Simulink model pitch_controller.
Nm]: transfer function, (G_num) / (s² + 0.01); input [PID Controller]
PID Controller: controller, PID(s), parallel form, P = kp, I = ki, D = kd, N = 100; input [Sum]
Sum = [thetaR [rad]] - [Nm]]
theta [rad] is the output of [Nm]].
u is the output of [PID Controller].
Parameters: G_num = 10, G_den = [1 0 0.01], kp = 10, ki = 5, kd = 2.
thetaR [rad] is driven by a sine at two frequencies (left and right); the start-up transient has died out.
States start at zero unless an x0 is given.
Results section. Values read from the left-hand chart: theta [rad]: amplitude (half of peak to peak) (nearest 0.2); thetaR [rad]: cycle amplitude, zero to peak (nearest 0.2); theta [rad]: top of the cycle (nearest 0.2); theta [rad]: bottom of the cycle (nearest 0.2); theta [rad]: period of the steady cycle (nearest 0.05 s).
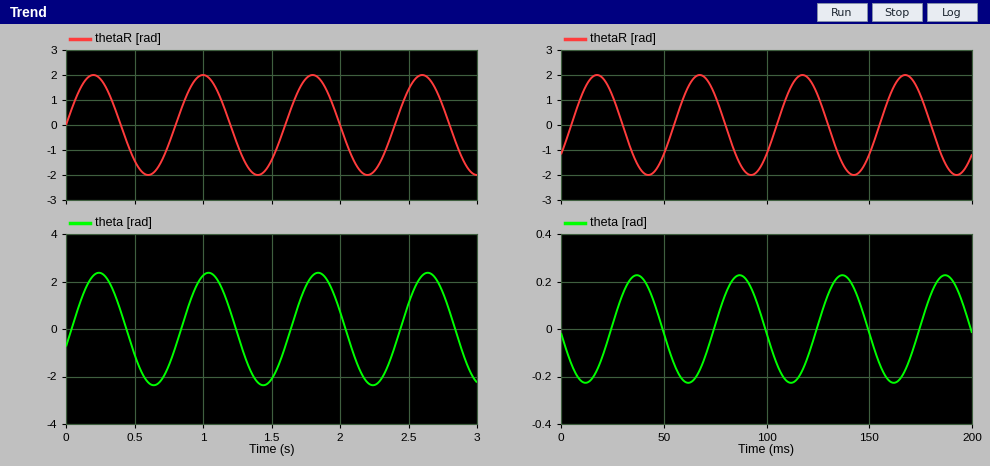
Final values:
2.4
2.0
2.4
-2.4
0.80 s
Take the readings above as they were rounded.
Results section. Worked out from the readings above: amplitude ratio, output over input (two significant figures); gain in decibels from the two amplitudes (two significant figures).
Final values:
1.2
1.6 dB
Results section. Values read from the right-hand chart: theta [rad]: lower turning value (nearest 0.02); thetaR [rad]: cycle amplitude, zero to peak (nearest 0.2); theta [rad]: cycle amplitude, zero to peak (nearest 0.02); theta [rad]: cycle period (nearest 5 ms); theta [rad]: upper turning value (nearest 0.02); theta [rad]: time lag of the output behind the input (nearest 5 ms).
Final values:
-0.22
2.0
0.22
50 ms
0.22
20 ms
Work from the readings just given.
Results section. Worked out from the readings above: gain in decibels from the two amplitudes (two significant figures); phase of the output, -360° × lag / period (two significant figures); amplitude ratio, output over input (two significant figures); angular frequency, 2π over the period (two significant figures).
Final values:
-19 dB
-140°
0.11
0.13 rad/ms
